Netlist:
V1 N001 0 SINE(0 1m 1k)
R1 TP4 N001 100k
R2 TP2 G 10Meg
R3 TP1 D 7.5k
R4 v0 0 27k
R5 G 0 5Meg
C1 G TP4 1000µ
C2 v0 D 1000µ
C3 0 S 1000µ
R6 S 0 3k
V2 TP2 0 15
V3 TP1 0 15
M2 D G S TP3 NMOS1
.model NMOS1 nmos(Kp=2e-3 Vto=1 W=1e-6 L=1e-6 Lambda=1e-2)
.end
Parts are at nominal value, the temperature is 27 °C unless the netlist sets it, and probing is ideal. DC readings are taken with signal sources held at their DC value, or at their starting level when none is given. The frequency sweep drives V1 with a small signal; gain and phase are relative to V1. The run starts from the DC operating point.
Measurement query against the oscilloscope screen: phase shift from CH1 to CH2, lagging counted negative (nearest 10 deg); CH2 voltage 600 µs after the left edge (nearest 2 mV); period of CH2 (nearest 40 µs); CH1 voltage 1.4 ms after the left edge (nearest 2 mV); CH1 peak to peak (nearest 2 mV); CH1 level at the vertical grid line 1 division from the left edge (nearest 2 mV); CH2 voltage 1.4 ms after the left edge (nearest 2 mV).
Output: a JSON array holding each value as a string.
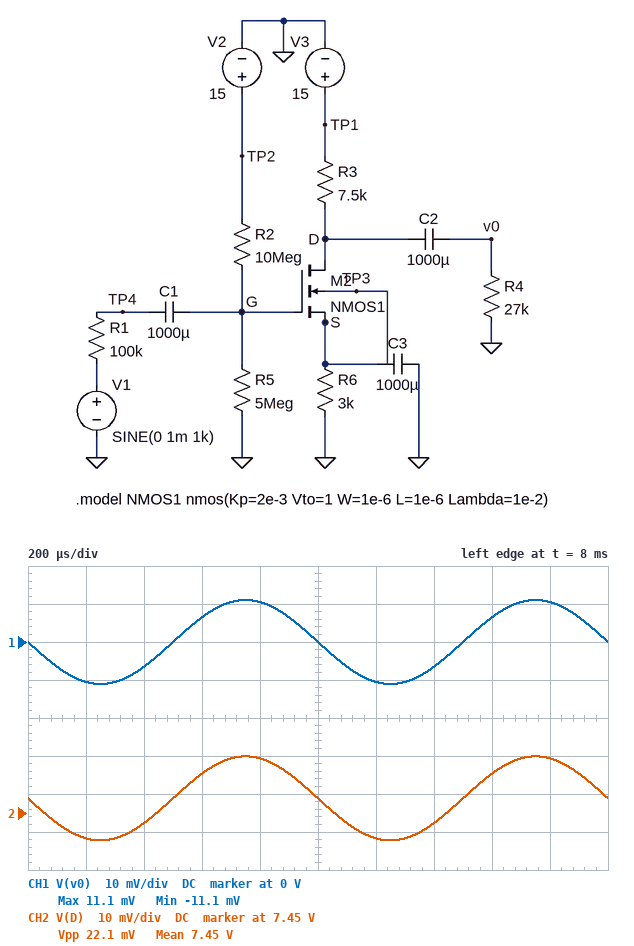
["0 deg", "7.460 V", "1.00 ms", "-6 mV", "22 mV", "-10 mV", "7.448 V"]
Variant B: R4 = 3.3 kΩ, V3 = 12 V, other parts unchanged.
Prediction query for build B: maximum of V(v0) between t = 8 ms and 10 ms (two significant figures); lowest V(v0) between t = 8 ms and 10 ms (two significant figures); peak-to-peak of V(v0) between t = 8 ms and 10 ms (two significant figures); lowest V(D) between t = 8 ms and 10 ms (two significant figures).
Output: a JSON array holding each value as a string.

["4.4 mV", "-4.4 mV", "8.8 mV", "4.5 V"]
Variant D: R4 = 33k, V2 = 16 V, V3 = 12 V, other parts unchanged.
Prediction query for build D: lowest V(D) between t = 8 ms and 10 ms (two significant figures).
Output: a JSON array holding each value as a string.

["3.9 V"]
